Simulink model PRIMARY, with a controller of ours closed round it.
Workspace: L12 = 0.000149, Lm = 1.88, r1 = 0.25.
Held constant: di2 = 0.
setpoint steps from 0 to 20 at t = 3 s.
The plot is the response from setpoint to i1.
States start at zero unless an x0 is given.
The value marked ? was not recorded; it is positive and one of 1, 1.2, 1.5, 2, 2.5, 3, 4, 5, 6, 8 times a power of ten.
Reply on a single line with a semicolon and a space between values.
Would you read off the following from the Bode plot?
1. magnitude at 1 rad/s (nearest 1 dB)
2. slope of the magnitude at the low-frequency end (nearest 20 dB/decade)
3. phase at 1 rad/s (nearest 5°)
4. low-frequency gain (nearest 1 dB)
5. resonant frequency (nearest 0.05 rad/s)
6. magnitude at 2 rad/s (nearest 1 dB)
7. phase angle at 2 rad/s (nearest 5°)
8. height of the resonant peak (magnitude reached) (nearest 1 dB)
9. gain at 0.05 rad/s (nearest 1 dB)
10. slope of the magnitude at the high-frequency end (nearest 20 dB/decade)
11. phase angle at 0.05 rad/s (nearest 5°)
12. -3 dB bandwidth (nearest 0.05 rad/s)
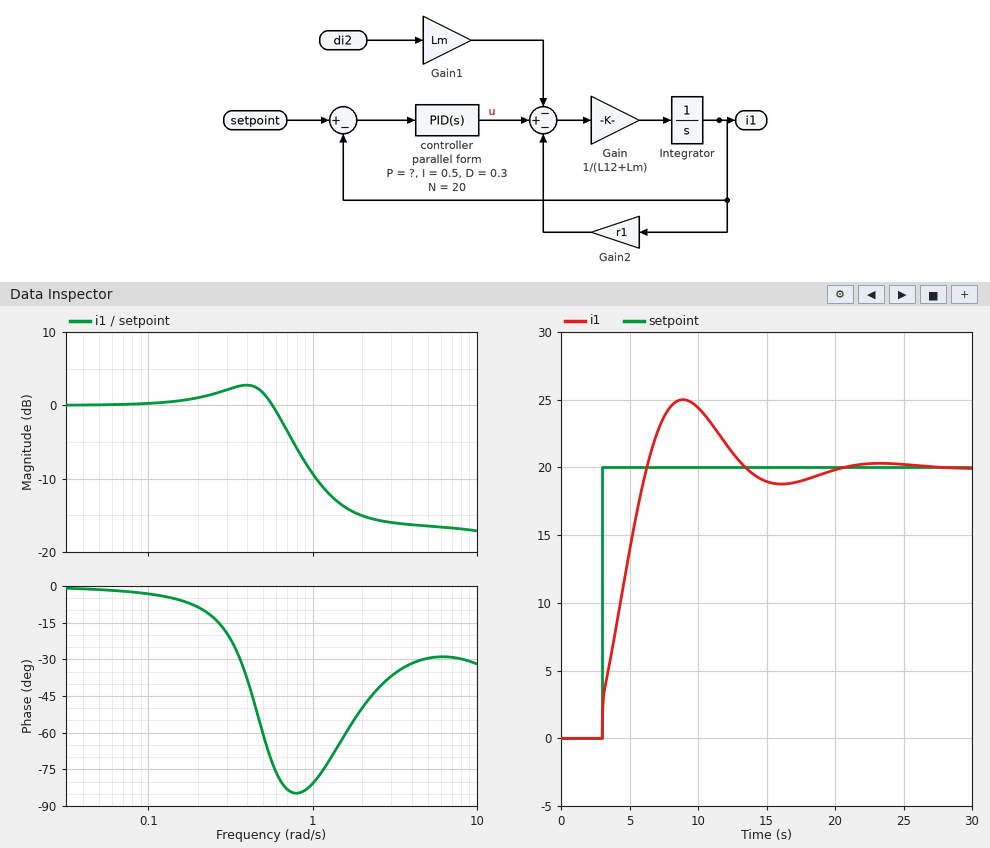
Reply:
-9 dB; 0 dB/decade; -80°; 0 dB; 0.40 rad/s; -15 dB; -50°; 3 dB; 0 dB; 0 dB/decade; 0°; 0.70 rad/s
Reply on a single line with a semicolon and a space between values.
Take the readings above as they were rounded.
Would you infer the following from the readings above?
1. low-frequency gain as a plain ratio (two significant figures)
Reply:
1.0
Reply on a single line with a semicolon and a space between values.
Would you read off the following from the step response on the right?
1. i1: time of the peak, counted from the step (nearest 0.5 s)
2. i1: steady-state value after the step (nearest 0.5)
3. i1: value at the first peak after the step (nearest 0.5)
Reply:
6.0 s; 20.0; 25.0
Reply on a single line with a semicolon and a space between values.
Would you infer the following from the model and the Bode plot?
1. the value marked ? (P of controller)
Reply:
0.6
